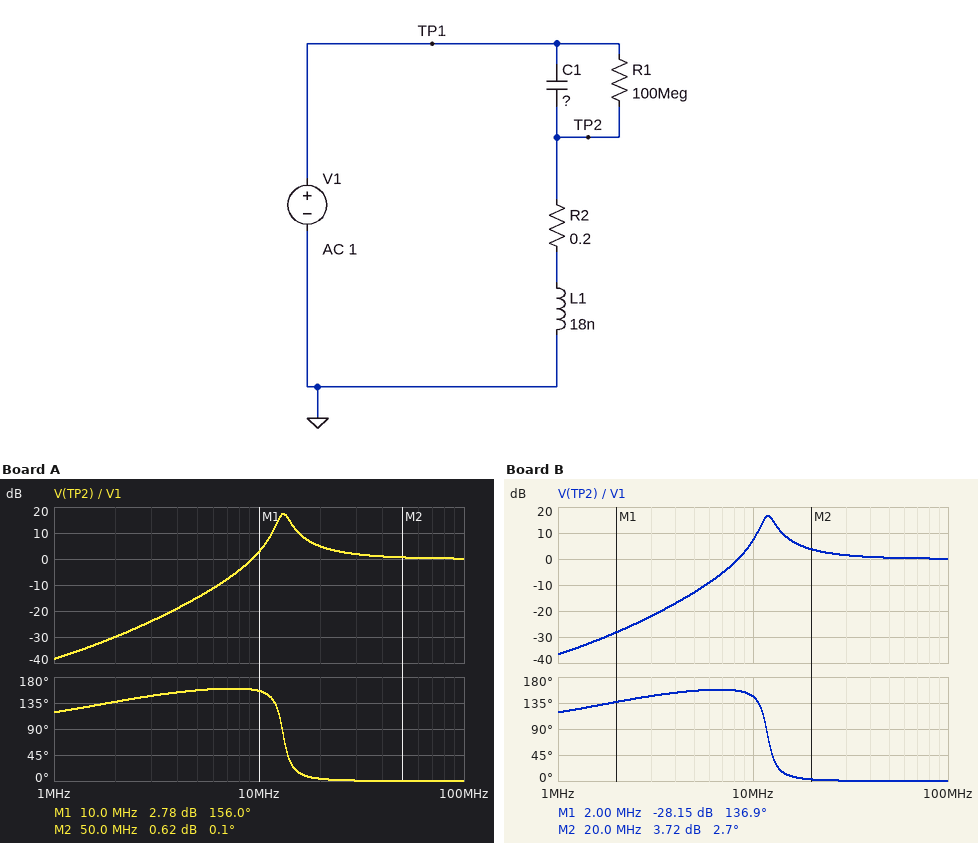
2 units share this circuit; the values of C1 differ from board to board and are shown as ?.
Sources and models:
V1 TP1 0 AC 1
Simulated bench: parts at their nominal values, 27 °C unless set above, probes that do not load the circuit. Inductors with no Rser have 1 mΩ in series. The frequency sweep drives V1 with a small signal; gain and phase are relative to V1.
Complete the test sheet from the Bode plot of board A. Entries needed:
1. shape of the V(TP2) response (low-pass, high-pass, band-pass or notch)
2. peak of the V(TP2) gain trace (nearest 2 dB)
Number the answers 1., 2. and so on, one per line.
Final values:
1. high-pass
2. 18 dB
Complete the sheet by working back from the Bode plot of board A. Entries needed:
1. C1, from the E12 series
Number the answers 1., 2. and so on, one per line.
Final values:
1. 8.2 nF
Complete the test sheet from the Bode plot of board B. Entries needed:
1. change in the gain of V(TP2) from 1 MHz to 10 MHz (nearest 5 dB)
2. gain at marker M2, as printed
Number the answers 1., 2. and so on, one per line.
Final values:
1. 45 dB
2. 3.72 dB
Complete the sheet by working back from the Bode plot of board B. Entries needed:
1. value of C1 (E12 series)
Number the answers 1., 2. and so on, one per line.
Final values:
1. 10 nF
